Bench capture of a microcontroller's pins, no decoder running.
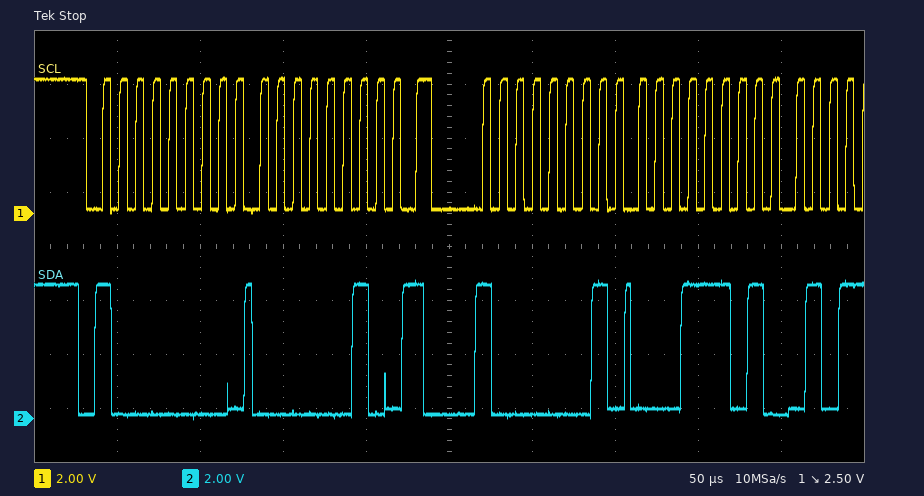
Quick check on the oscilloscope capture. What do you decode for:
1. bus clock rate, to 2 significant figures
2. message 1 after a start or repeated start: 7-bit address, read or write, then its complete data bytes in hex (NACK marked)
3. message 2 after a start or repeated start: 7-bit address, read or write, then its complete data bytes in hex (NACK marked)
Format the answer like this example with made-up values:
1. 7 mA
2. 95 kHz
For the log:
1. 100 kHz
2. 0x40 write: 02
3. 0x40 read: 1D
